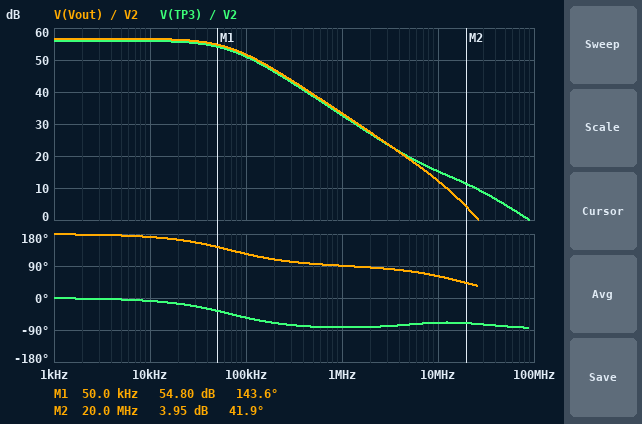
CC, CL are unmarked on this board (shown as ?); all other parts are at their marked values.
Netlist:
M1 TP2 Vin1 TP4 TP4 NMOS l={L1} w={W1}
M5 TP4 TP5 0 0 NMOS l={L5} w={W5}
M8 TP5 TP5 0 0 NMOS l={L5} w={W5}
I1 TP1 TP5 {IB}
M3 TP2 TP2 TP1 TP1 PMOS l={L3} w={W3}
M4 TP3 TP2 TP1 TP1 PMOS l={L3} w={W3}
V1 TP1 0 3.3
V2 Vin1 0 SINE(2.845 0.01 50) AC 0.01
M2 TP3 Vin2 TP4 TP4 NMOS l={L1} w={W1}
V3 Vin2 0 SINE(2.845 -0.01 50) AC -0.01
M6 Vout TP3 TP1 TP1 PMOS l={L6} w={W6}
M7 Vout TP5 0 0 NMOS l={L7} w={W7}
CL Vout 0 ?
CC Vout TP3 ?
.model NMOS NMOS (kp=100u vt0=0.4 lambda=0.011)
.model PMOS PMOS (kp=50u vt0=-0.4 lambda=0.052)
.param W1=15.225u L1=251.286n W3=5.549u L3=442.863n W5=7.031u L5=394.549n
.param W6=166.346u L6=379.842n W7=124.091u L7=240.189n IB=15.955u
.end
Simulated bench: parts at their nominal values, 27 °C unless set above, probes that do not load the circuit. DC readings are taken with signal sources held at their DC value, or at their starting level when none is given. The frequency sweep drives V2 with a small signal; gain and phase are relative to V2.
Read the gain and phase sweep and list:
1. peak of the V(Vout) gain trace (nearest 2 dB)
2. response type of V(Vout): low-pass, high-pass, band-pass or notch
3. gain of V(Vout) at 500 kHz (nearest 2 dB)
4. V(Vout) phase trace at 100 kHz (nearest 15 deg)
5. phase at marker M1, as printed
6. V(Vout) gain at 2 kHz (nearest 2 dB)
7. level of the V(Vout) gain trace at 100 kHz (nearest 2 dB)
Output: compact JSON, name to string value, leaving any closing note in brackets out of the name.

{"peak of the V(Vout) gain trace": "56 dB", "response type of V(Vout): low-pass, high-pass, band-pass or notch": "low-pass", "gain of V(Vout) at 500 kHz": "40 dB", "V(Vout) phase trace at 100 kHz": "120 deg", "phase at marker M1, as printed": "143.6 deg", "V(Vout) gain at 2 kHz": "56 dB", "level of the V(Vout) gain trace at 100 kHz": "52 dB"}
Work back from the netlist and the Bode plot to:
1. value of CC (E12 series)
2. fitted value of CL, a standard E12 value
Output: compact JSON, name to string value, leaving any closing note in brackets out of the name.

{"value of CC": "560 fF", "fitted value of CL, a standard E12 value": "68 pF"}
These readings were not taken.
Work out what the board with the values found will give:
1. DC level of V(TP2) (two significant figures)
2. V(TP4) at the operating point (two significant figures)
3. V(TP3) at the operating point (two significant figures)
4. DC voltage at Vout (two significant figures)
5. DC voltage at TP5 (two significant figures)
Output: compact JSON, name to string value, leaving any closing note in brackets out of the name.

{"DC level of V(TP2)": "2.7 V", "V(TP4) at the operating point": "2.4 V", "V(TP3) at the operating point": "2.7 V", "DC voltage at Vout": "61 mV", "DC voltage at TP5": "530 mV"}
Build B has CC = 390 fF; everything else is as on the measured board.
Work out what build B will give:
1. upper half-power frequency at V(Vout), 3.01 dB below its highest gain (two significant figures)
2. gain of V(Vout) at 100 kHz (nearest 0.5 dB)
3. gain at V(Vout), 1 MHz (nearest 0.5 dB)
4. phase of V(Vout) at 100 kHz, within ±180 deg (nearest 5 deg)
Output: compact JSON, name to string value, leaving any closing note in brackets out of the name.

{"upper half-power frequency at V(Vout), 3.01 dB below its highest gain": "98 kHz", "gain of V(Vout) at 100 kHz": "53.5 dB", "gain at V(Vout), 1 MHz": "36.5 dB", "phase of V(Vout) at 100 kHz, within ±180 deg": "135 deg"}
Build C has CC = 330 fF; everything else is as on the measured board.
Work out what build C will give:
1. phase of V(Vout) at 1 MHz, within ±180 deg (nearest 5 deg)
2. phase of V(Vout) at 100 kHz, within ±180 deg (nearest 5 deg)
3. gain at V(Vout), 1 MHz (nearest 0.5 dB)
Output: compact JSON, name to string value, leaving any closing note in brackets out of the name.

{"phase of V(Vout) at 1 MHz, within ±180 deg": "95 deg", "phase of V(Vout) at 100 kHz, within ±180 deg": "140 deg", "gain at V(Vout), 1 MHz": "38.0 dB"}
